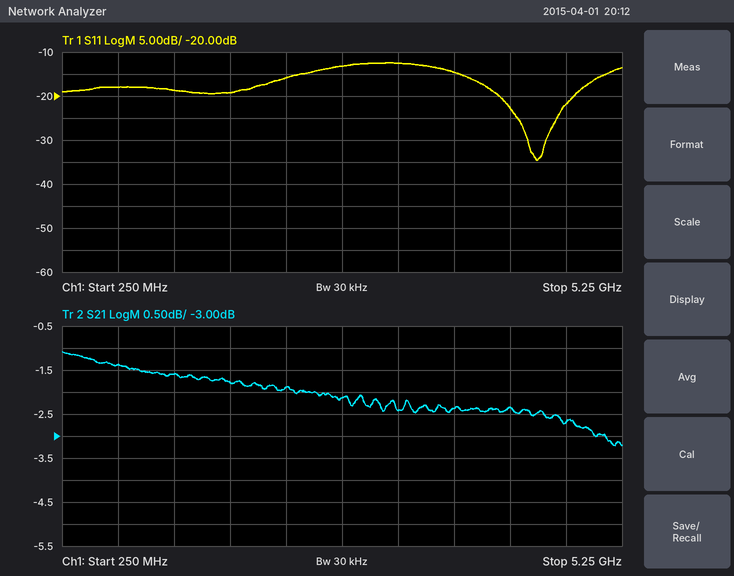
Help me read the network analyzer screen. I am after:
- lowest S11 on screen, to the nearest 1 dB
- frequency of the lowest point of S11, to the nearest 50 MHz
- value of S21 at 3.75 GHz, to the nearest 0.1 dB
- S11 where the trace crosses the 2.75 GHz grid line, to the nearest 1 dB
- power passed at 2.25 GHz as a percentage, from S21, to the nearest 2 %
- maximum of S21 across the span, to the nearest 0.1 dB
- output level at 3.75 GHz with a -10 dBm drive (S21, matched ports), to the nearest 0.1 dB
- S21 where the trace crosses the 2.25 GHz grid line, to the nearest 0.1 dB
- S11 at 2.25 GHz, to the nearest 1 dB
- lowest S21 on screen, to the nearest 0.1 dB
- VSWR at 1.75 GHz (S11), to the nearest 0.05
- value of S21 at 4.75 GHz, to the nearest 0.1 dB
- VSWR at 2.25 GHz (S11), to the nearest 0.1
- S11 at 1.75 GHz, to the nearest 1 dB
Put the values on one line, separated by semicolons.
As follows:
-35 dB; 4.50 GHz; -2.4 dB; -13 dB; 64 %; -1.1 dB; -12.4 dBm; -1.9 dB; -16 dB; -3.2 dB; 1.25; -2.7 dB; 1.4; -19 dB
